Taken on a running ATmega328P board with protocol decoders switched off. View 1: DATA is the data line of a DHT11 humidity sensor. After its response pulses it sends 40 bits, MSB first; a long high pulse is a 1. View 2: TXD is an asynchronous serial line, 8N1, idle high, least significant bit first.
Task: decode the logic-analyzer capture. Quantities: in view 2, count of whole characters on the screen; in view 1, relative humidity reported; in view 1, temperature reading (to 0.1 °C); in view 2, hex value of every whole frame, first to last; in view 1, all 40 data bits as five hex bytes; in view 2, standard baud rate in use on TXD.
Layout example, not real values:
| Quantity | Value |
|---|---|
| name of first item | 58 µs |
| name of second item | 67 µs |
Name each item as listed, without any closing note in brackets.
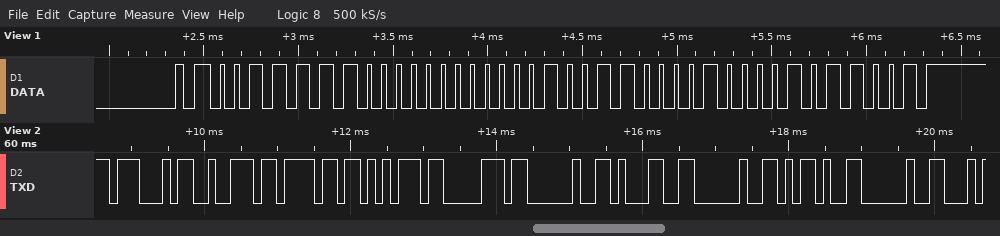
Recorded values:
| Quantity | Value |
|---|---|
| in view 2, count of whole characters on the screen | 10 |
| in view 1, relative humidity reported | 62 % |
| in view 1, temperature reading | 19.8 °C |
| in view 2, hex value of every whole frame, first to last | 0x47 0x72 0x6F 0x75 0x70 0x20 0x31 0x20 0x2D 0x20 |
| in view 1, all 40 data bits as five hex bytes | 3E 00 13 08 59 |
| in view 2, standard baud rate in use on TXD | 9600 baud |
